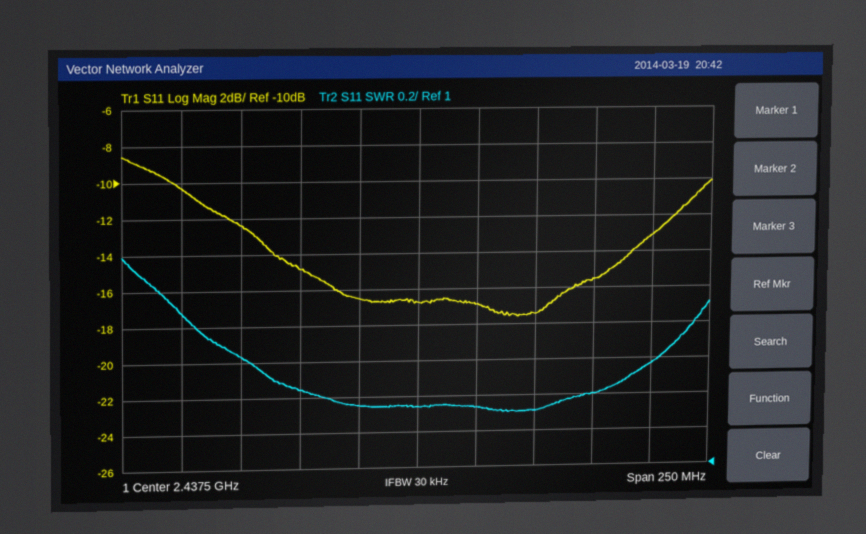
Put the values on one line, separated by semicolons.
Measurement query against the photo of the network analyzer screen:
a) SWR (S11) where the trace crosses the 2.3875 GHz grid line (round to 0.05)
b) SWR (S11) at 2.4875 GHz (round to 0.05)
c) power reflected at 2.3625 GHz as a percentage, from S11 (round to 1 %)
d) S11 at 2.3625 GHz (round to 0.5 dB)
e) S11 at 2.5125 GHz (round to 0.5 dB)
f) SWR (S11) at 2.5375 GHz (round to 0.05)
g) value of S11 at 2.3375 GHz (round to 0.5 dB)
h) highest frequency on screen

1.45; 1.30; 6 %; -12.5 dB; -15.5 dB; 1.55; -10.5 dB; 2.5625 GHz
